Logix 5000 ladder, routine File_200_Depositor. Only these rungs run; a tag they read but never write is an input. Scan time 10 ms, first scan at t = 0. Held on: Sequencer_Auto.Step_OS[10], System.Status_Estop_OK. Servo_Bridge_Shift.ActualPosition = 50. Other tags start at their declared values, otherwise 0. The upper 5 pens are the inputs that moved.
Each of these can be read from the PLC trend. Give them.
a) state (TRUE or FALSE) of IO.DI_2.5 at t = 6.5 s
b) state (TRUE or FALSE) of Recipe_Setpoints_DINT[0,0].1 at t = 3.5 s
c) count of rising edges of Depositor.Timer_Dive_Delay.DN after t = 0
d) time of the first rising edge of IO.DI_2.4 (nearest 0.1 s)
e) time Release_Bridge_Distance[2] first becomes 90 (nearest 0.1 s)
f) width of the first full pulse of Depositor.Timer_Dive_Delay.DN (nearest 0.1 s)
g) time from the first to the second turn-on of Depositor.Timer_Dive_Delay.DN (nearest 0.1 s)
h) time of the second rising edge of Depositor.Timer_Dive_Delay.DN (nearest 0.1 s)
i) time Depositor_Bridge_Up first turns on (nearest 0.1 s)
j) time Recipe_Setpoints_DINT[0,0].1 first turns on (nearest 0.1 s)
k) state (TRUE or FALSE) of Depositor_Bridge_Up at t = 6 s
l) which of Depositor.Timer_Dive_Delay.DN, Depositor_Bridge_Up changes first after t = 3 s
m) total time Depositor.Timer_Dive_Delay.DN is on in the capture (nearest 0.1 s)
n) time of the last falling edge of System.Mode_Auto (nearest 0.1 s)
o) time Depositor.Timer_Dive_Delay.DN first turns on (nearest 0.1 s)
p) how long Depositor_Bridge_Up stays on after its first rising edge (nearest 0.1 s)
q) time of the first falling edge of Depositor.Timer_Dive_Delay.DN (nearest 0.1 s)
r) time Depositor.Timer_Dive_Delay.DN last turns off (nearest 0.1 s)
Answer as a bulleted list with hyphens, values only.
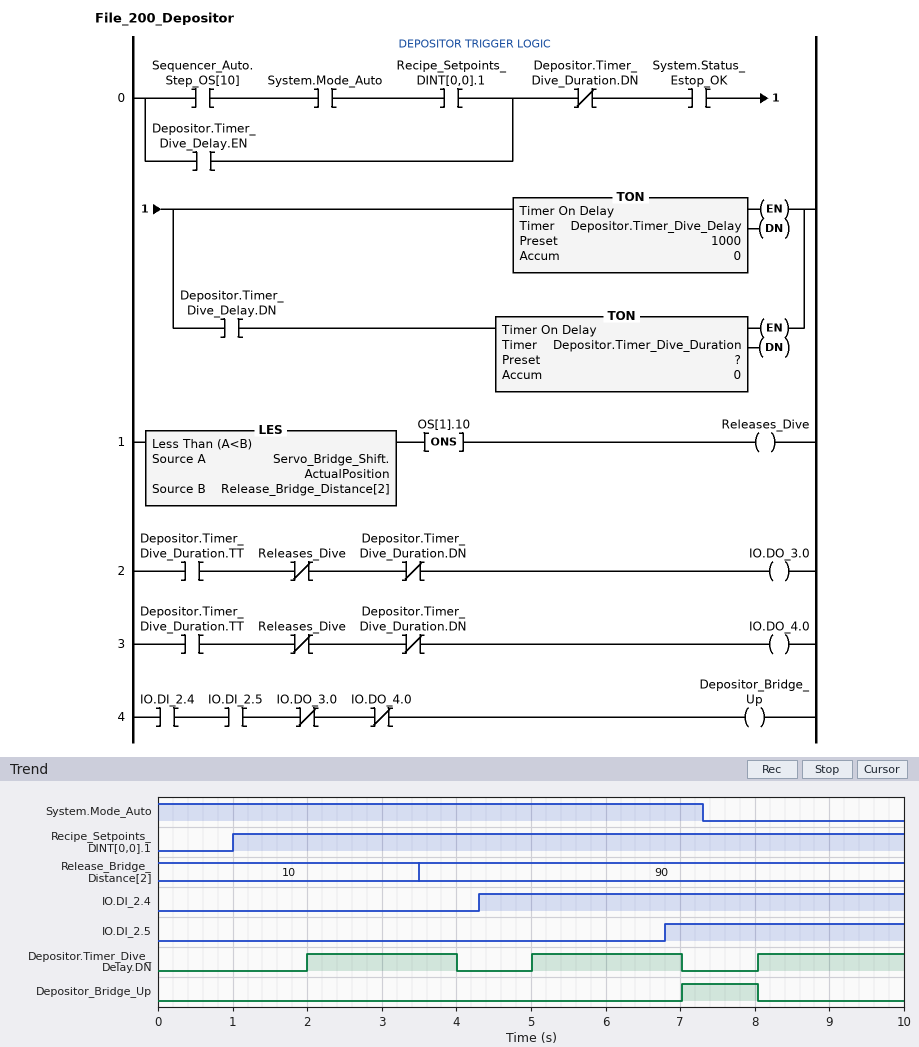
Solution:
- FALSE
- TRUE
- 3
- 4.3 s
- 3.5 s
- 2.0 s
- 3.0 s
- 5.0 s
- 7.0 s
- 1.0 s
- FALSE
- Depositor.Timer_Dive_Delay.DN
- 6.0 s
- 7.3 s
- 2.0 s
- 1.0 s
- 4.0 s
- 7.0 s
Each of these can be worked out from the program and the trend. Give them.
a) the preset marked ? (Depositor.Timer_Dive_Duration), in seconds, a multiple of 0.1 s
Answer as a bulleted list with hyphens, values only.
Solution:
- 2.0 s
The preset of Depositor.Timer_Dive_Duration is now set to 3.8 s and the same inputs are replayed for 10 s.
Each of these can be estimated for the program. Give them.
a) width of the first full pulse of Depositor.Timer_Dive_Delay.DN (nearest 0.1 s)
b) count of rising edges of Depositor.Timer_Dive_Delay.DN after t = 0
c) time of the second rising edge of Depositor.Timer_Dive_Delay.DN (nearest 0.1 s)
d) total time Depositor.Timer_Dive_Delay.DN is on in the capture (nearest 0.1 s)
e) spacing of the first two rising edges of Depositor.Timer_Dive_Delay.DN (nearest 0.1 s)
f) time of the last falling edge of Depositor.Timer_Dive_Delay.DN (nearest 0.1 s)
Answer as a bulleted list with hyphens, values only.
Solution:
- 3.8 s
- 2
- 6.8 s
- 7.0 s
- 4.8 s
- 5.8 s
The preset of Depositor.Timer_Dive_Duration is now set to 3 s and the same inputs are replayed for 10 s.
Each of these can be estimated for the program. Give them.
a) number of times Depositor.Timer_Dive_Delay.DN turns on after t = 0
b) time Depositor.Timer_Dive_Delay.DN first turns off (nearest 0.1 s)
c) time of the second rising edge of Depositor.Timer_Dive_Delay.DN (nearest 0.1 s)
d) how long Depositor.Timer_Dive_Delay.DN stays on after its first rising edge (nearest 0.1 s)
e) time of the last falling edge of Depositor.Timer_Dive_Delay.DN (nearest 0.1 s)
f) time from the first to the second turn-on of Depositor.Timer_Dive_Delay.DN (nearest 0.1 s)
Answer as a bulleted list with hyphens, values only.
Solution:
- 2
- 5.0 s
- 6.0 s
- 3.0 s
- 9.0 s
- 4.0 s
